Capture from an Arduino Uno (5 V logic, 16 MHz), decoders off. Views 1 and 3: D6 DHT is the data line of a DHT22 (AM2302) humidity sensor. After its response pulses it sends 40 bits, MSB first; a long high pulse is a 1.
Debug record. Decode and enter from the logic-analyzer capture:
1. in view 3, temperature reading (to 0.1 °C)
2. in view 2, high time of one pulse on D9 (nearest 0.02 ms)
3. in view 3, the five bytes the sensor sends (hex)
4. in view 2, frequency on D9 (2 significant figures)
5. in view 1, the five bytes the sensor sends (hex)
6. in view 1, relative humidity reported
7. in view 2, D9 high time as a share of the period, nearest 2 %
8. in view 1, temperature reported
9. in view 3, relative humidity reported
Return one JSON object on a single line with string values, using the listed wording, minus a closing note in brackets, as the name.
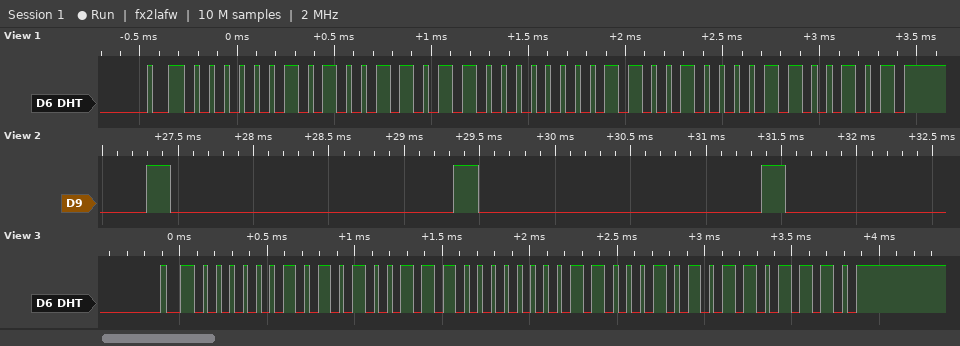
{"in view 3, temperature reading": "19.7 °C", "in view 2, high time of one pulse on D9": "0.16 ms", "in view 3, the five bytes the sensor sends": "02 A7 00 C5 6E", "in view 2, frequency on D9": "490 Hz", "in view 1, the five bytes the sensor sends": "02 9B 00 C8 65", "in view 1, relative humidity reported": "66.7 %", "in view 2, D9 high time as a share of the period, nearest 2 %": "8 %", "in view 1, temperature reported": "20.0 °C", "in view 3, relative humidity reported": "67.9 %"}
